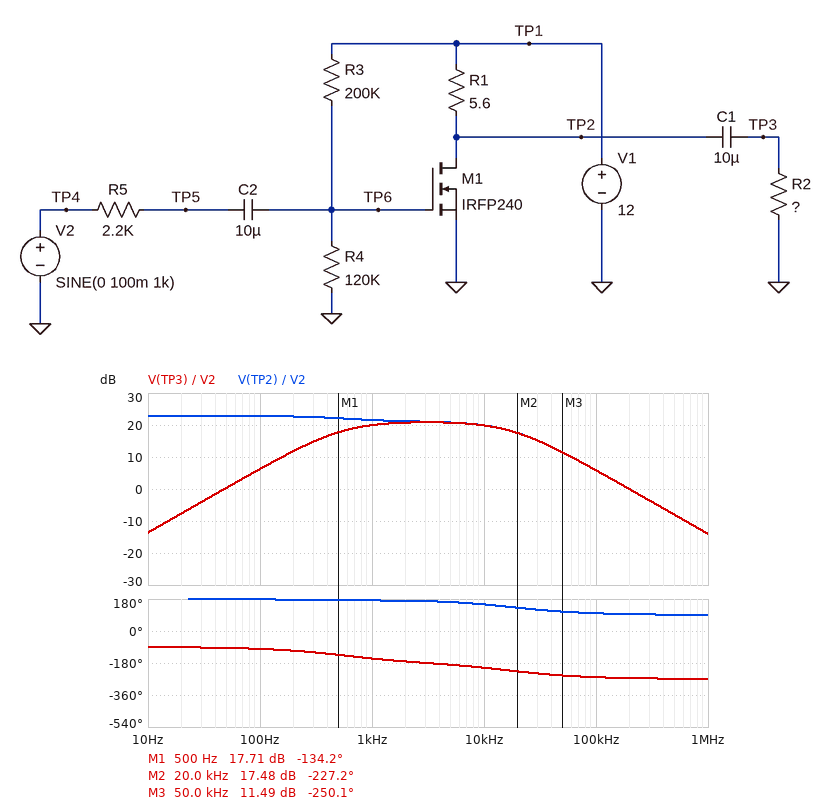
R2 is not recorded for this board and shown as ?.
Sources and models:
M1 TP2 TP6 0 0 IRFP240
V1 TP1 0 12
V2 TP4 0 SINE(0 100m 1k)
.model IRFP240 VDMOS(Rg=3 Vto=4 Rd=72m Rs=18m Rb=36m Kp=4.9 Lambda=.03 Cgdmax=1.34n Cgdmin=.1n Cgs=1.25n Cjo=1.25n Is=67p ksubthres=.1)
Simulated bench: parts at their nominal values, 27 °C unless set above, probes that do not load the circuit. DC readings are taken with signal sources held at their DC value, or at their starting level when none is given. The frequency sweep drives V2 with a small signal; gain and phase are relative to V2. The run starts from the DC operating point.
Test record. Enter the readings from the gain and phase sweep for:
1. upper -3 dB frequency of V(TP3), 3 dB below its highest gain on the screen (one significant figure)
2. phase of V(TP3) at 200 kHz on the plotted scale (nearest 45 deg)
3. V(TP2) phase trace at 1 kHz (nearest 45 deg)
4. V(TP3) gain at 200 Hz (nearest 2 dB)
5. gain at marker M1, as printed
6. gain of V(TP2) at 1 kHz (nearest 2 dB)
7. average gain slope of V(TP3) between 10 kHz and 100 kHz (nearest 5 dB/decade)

20 kHz
-270 deg
180 deg
12 dB
17.71 dB
22 dB
-15 dB/decade
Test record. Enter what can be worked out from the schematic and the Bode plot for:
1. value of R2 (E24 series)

24 Ω
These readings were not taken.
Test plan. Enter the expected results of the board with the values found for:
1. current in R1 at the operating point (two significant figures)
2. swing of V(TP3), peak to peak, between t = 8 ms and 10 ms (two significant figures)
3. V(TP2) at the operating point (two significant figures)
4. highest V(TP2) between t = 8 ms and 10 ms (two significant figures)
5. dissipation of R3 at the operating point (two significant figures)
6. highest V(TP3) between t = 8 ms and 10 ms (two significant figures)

720 mA
2.0 V
8.0 V
9.1 V
280 µW
970 mV
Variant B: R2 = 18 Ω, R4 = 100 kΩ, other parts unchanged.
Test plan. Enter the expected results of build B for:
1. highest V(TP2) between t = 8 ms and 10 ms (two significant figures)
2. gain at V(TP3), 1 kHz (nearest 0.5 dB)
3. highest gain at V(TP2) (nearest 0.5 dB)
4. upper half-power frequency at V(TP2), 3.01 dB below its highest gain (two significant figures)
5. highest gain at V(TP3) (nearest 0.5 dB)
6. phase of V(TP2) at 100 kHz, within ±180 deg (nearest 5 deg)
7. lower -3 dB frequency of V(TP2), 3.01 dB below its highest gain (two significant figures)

12 V
-2.0 dB
2.0 dB
19 kHz
-0.5 dB
115 deg
230 mHz
